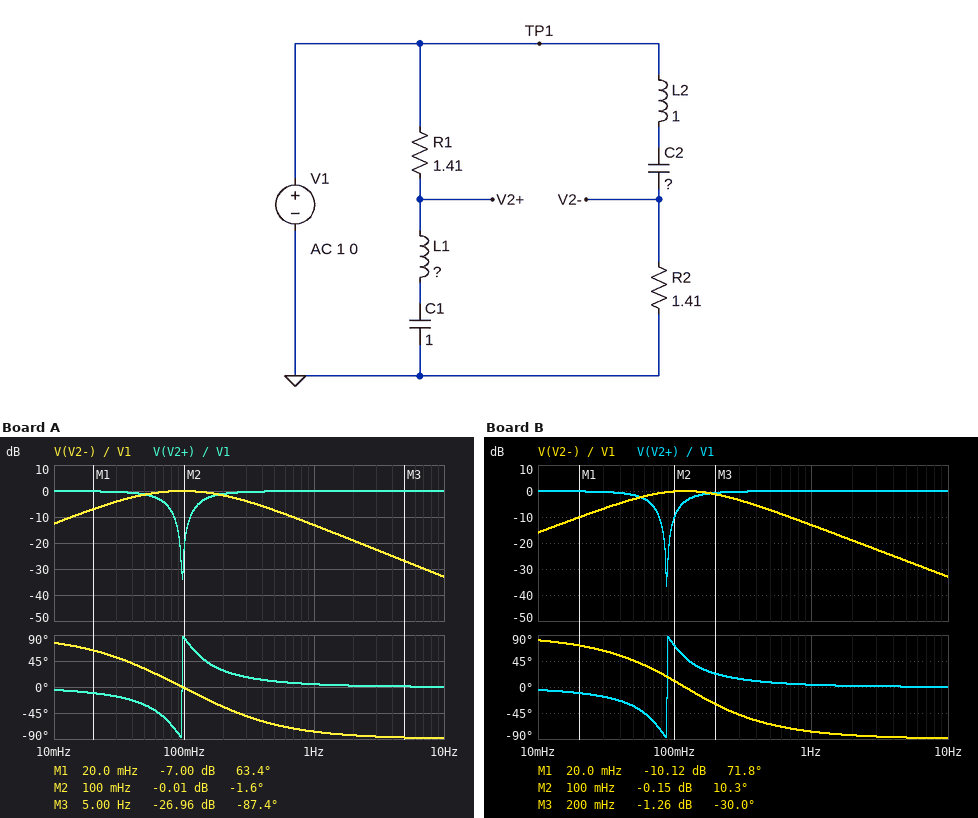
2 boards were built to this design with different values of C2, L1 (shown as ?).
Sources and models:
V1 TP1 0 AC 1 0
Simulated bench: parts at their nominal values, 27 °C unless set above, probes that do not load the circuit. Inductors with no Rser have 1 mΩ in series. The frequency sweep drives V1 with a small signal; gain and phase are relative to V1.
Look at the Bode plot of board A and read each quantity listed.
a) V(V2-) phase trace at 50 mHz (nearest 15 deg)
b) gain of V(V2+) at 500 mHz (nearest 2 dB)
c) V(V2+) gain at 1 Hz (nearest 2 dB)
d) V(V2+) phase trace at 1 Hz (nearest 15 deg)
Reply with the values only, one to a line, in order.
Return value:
30 deg
0 dB
0 dB
0 deg
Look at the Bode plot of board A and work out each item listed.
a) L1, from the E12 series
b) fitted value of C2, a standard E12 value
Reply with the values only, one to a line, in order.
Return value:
2.7 H
2.7 F
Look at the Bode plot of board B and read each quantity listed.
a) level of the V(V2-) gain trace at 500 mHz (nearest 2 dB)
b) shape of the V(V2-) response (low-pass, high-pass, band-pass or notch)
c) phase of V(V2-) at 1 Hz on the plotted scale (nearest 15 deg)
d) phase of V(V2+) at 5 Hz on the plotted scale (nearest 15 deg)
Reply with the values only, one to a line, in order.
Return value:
-8 dB
band-pass
-75 deg
0 deg
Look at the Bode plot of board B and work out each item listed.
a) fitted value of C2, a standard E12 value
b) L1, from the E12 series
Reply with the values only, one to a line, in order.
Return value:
1.8 F
3.3 H
